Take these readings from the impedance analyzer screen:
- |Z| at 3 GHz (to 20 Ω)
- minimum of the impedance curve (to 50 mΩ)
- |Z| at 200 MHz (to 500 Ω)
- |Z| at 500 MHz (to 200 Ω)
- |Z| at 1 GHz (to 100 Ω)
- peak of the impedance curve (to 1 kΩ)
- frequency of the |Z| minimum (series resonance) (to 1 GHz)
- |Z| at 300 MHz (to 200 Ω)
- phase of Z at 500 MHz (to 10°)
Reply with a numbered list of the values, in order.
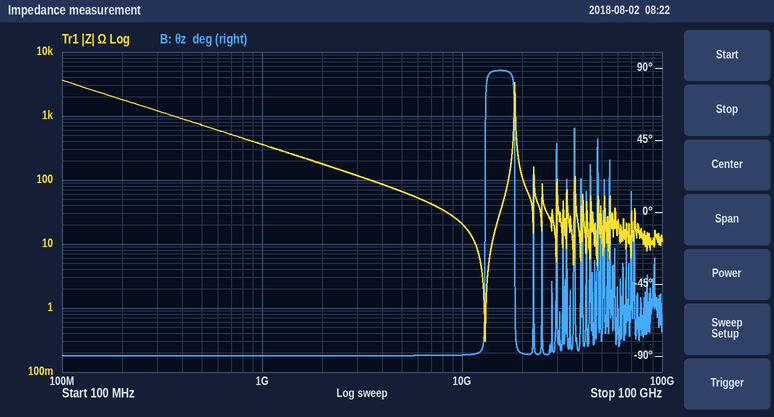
1. 120 Ω
2. 300 mΩ
3. 2.0 kΩ
4. 800 Ω
5. 400 Ω
6. 4 kΩ
7. 13 GHz
8. 1.2 kΩ
9. -90°
